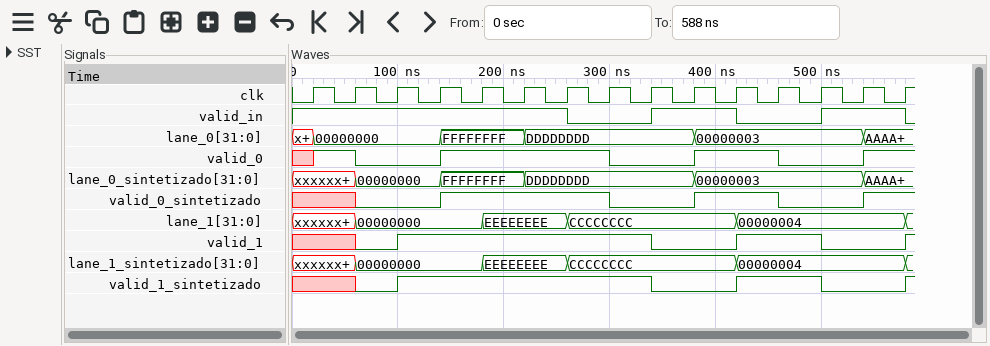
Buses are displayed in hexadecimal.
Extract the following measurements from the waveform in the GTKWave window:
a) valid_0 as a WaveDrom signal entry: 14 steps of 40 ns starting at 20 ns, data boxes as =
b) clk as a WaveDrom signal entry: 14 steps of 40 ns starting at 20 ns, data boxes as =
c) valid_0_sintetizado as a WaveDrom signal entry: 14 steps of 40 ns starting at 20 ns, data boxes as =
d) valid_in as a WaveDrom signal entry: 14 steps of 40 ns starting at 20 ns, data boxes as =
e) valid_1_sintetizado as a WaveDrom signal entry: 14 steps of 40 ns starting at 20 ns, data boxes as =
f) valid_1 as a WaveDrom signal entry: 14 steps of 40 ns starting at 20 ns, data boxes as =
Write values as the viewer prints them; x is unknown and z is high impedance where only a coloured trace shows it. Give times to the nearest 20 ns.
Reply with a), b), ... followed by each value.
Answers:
a) {name: 'valid_0', wave: '10.1...0.1.0.1'}
b) {name: 'clk', wave: 'p.............'}
c) {name: 'valid_0_sintetizado', wave: 'x0.1...0.1.0.1'}
d) {name: 'valid_in', wave: '1.....0.1.0.1.'}
e) {name: 'valid_1_sintetizado', wave: 'x01.....0.1.0.'}
f) {name: 'valid_1', wave: 'x01.....0.1.0.'}
